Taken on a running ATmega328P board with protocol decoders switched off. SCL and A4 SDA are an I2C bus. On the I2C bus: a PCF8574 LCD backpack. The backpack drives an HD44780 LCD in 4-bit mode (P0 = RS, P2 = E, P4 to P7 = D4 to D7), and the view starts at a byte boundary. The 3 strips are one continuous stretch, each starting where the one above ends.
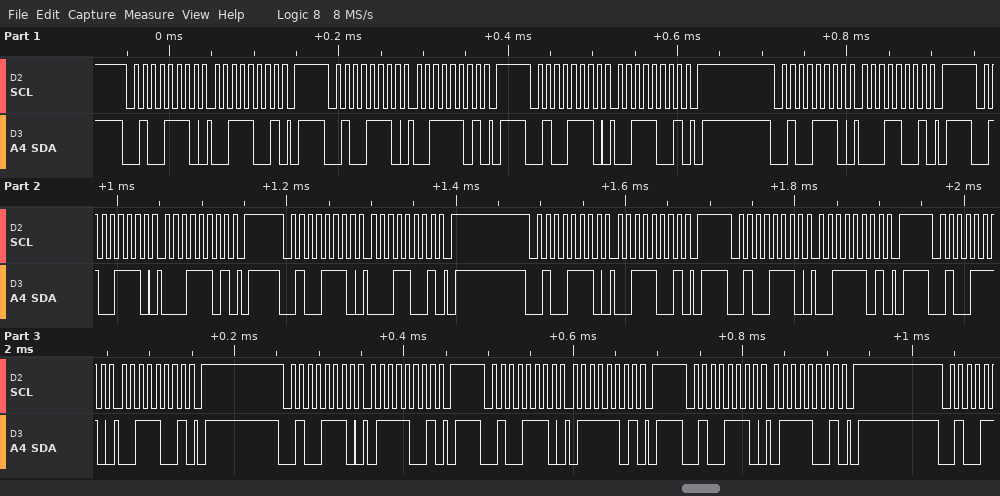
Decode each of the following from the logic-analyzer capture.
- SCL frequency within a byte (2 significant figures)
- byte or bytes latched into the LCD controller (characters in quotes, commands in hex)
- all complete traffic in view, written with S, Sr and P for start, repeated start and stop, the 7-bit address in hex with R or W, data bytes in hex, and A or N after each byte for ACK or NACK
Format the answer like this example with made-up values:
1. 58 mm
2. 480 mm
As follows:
1. 100 kHz
2. '1' '7'
3. S 27W A 39 A P S 27W A 3D A P S 27W A 39 A P S 27W A 19 A P S 27W A 1D A P S 27W A 19 A P S 27W A 39 A P S 27W A 3D A P S 27W A 39 A P S 27W A 79 A P S 27W A 7D A P S 27W A 79 A P
